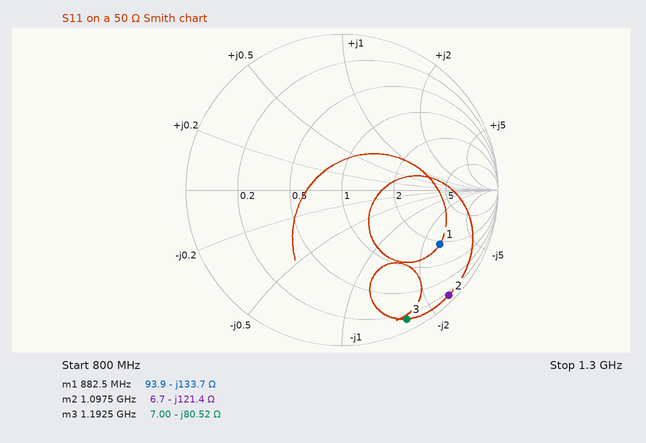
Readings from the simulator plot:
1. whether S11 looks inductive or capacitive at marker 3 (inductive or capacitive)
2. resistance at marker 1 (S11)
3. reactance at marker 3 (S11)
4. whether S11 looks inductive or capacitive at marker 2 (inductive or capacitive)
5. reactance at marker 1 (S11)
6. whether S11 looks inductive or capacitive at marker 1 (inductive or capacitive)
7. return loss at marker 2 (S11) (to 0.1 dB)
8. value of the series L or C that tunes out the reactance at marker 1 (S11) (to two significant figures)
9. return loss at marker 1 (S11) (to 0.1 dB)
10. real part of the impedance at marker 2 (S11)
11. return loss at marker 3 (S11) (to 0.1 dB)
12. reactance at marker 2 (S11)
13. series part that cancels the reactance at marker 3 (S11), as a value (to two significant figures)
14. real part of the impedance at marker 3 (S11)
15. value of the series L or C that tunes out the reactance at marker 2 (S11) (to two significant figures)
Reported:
capacitive
93.9 Ω
-80.52 Ω
capacitive
-133.7 Ω
capacitive
0.3 dB
24 nH
2.9 dB
6.7 Ω
0.7 dB
-121.4 Ω
11 nH
7.00 Ω
18 nH
